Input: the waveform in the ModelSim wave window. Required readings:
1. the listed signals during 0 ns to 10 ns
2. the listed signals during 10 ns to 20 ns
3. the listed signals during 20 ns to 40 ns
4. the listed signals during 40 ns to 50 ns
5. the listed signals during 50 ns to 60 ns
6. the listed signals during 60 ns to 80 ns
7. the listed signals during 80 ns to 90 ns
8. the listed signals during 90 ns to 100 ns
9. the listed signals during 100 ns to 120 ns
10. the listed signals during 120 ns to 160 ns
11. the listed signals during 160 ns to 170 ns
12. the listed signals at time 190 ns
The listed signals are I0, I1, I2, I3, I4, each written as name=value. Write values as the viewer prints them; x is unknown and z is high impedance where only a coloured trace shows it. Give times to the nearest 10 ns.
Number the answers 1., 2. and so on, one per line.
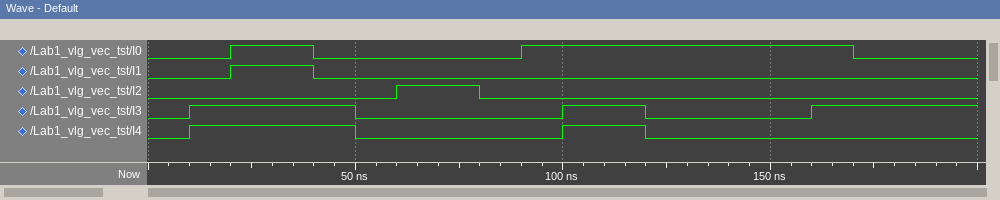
1. I0=0, I1=0, I2=0, I3=0, I4=0
2. I0=0, I1=0, I2=0, I3=1, I4=1
3. I0=1, I1=1, I2=0, I3=1, I4=1
4. I0=0, I1=0, I2=0, I3=1, I4=1
5. I0=0, I1=0, I2=0, I3=0, I4=0
6. I0=0, I1=0, I2=1, I3=0, I4=0
7. I0=0, I1=0, I2=0, I3=0, I4=0
8. I0=1, I1=0, I2=0, I3=0, I4=0
9. I0=1, I1=0, I2=0, I3=1, I4=1
10. I0=1, I1=0, I2=0, I3=0, I4=0
11. I0=1, I1=0, I2=0, I3=1, I4=0
12. I0=0, I1=0, I2=0, I3=1, I4=0
